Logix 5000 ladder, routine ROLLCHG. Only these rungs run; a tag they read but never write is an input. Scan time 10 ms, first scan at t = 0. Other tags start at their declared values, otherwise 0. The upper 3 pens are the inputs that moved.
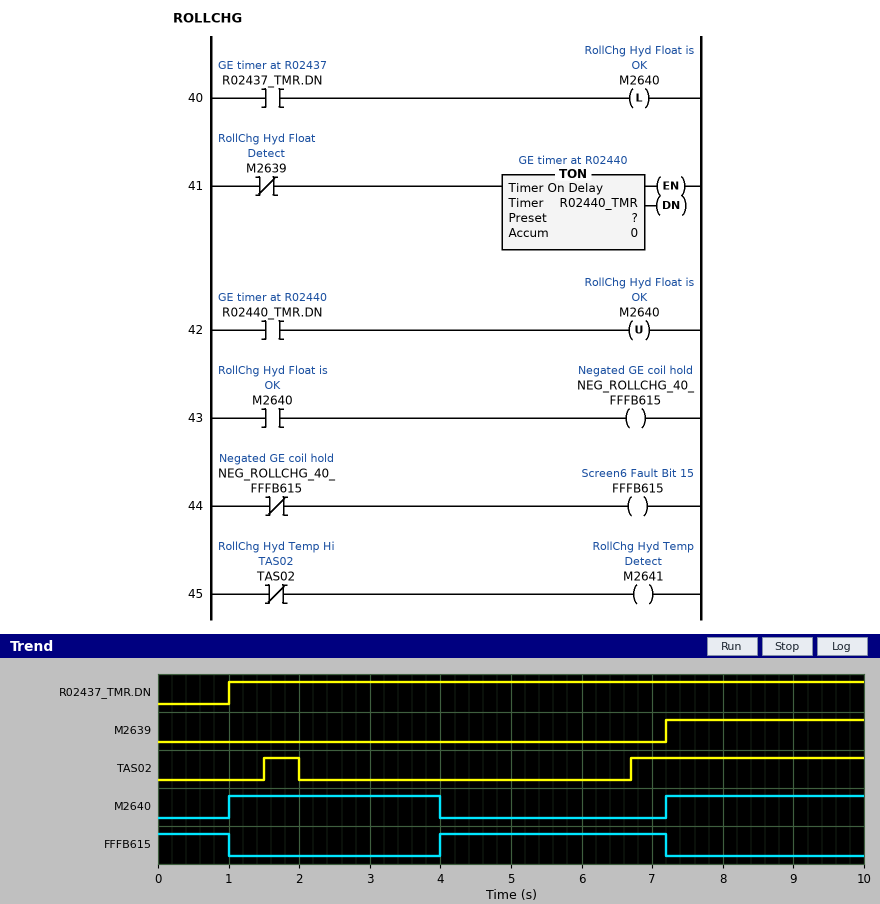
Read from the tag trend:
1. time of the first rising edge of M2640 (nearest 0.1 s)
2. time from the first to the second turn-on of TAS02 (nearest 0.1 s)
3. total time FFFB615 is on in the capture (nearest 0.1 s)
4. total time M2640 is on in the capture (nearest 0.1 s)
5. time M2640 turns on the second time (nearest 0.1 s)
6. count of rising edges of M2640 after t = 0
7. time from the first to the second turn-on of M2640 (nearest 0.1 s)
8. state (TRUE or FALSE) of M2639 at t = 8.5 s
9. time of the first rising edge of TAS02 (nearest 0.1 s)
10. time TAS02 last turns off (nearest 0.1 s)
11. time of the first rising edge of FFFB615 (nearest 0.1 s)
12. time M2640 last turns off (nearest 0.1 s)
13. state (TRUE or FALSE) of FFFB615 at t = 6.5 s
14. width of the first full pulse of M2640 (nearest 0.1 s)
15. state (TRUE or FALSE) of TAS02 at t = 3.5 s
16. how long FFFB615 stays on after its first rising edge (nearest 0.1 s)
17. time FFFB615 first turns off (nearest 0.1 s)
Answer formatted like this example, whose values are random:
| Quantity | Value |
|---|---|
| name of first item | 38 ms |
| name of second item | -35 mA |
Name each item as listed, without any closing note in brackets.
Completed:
| Quantity | Value |
|---|---|
| time of the first rising edge of M2640 | 1.0 s |
| time from the first to the second turn-on of TAS02 | 5.2 s |
| total time FFFB615 is on in the capture | 4.2 s |
| total time M2640 is on in the capture | 5.8 s |
| time M2640 turns on the second time | 7.2 s |
| count of rising edges of M2640 after t = 0 | 2 |
| time from the first to the second turn-on of M2640 | 6.2 s |
| state (TRUE or FALSE) of M2639 at t = 8.5 s | TRUE |
| time of the first rising edge of TAS02 | 1.5 s |
| time TAS02 last turns off | 2.0 s |
| time of the first rising edge of FFFB615 | 4.0 s |
| time M2640 last turns off | 4.0 s |
| state (TRUE or FALSE) of FFFB615 at t = 6.5 s | TRUE |
| width of the first full pulse of M2640 | 3.0 s |
| state (TRUE or FALSE) of TAS02 at t = 3.5 s | FALSE |
| how long FFFB615 stays on after its first rising edge | 3.2 s |
| time FFFB615 first turns off | 1.0 s |
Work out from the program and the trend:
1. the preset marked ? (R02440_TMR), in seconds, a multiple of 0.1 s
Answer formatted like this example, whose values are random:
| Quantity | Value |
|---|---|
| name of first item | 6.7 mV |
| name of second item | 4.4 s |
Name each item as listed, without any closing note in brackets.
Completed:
| Quantity | Value |
|---|---|
| the preset marked ? (R02440_TMR), in seconds, a multiple of 0.1 s | 4.0 s |
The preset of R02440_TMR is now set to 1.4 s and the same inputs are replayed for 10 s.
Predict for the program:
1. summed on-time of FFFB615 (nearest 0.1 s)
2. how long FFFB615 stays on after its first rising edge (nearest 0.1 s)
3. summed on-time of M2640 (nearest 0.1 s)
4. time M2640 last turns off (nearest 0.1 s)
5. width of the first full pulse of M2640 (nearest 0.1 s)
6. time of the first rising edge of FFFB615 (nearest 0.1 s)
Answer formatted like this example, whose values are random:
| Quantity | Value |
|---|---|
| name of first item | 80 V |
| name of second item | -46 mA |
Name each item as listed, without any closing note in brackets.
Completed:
| Quantity | Value |
|---|---|
| summed on-time of FFFB615 | 6.8 s |
| how long FFFB615 stays on after its first rising edge | 5.8 s |
| summed on-time of M2640 | 3.2 s |
| time M2640 last turns off | 1.4 s |
| width of the first full pulse of M2640 | 0.4 s |
| time of the first rising edge of FFFB615 | 1.4 s |
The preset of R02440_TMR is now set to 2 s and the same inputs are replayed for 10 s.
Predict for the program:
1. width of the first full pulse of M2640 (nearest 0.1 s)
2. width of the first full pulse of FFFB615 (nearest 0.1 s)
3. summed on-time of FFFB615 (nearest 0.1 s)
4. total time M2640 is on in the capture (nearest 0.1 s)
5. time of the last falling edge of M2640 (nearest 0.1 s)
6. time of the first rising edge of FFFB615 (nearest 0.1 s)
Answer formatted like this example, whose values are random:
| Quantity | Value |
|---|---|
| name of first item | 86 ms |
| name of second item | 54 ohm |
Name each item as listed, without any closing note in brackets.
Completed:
| Quantity | Value |
|---|---|
| width of the first full pulse of M2640 | 1.0 s |
| width of the first full pulse of FFFB615 | 5.2 s |
| summed on-time of FFFB615 | 6.2 s |
| total time M2640 is on in the capture | 3.8 s |
| time of the last falling edge of M2640 | 2.0 s |
| time of the first rising edge of FFFB615 | 2.0 s |
